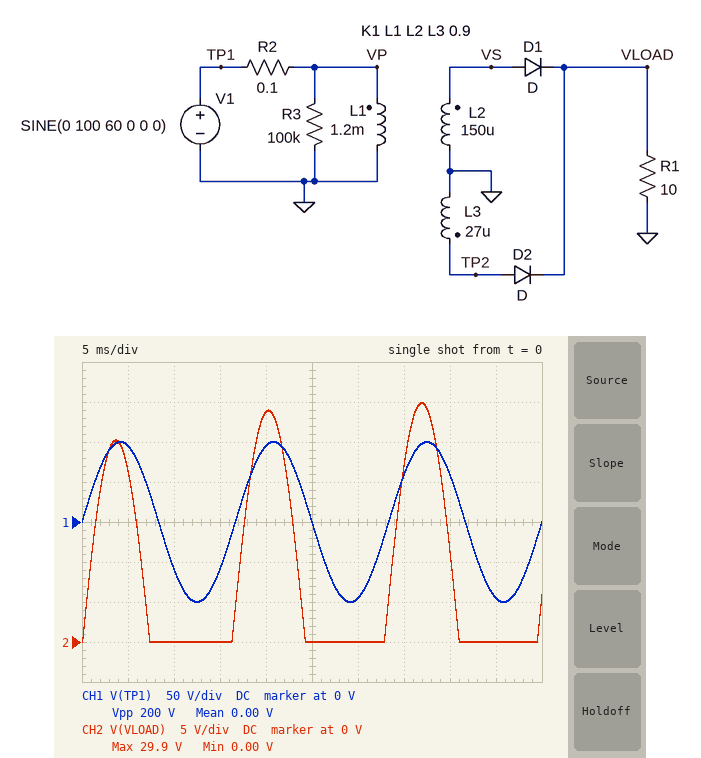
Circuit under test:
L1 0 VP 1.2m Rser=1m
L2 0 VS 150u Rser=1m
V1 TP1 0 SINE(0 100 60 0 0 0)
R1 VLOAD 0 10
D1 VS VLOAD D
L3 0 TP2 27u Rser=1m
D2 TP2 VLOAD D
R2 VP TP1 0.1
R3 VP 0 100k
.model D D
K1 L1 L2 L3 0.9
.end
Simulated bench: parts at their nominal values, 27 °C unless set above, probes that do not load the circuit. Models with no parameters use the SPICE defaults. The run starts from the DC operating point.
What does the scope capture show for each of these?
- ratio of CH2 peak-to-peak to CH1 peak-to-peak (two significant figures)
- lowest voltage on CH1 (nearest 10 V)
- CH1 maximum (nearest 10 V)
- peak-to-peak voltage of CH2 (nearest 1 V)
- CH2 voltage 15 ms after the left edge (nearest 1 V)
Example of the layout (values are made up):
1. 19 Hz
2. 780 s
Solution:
1. 0.15
2. -100 V
3. 100 V
4. 30 V
5. 0 V
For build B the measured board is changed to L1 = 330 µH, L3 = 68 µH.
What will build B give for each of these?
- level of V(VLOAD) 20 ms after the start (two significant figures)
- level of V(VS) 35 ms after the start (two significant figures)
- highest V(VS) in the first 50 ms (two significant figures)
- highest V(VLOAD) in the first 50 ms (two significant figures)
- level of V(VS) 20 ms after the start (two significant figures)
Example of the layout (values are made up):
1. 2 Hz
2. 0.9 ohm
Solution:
1. 43 V
2. 45 V
3. 47 V
4. 46 V
5. 44 V
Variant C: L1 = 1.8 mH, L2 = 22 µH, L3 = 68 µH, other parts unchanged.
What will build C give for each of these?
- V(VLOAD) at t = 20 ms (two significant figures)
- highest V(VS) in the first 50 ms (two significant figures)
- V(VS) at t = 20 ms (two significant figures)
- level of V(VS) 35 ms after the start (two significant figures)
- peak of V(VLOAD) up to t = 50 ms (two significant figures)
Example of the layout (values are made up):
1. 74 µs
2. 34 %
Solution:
1. 15 V
2. 9.7 V
3. 9.2 V
4. 6.7 V
5. 16 V
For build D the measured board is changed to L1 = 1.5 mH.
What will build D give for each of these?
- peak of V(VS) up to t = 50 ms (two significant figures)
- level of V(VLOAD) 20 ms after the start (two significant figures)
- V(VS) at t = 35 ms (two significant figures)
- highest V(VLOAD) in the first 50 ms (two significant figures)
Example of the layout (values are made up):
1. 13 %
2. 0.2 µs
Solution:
1. 28 V
2. 26 V
3. 20 V
4. 27 V
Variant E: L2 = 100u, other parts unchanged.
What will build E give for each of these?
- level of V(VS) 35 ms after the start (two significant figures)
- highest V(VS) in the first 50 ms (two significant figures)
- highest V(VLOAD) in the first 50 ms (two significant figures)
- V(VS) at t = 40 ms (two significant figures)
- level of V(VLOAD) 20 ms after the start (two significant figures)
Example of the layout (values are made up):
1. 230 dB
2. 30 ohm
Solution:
1. 19 V
2. 25 V
3. 24 V
4. 9.9 V
5. 23 V
